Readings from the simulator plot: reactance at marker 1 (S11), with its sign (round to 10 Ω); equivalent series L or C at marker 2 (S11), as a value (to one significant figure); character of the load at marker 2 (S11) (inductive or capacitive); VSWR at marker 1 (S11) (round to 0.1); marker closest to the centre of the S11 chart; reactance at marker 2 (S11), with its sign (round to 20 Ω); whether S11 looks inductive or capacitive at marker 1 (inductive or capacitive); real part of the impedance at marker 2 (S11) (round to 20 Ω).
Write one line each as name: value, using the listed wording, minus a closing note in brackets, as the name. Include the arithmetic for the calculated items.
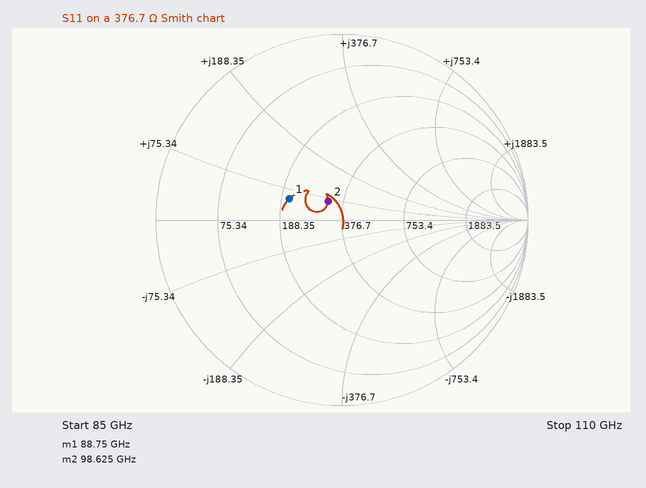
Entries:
reactance at marker 1 (S11), with its sign: +50 Ω
equivalent series L or C at marker 2 (S11), as a value: L = 60 Ω/(2π × 98.625 GHz) ≈ 96.8 pH, so 100 pH to one significant figure
character of the load at marker 2 (S11): inductive
VSWR at marker 1 (S11): 1.9
marker closest to the centre of the S11 chart: marker 2
reactance at marker 2 (S11), with its sign: +60 Ω
whether S11 looks inductive or capacitive at marker 1: inductive
real part of the impedance at marker 2 (S11): 320 Ω
